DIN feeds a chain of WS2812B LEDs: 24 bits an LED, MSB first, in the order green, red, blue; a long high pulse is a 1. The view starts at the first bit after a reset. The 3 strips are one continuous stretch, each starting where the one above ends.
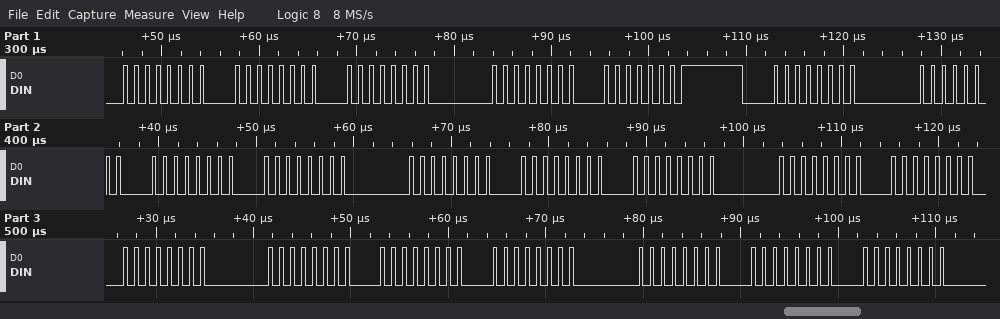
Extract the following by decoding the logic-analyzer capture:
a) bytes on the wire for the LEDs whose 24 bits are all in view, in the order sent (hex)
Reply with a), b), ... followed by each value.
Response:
a) 00 00 00 00 01 00 00 00 00 00 00 00 00 00 00 00 00 00 00 00 00
